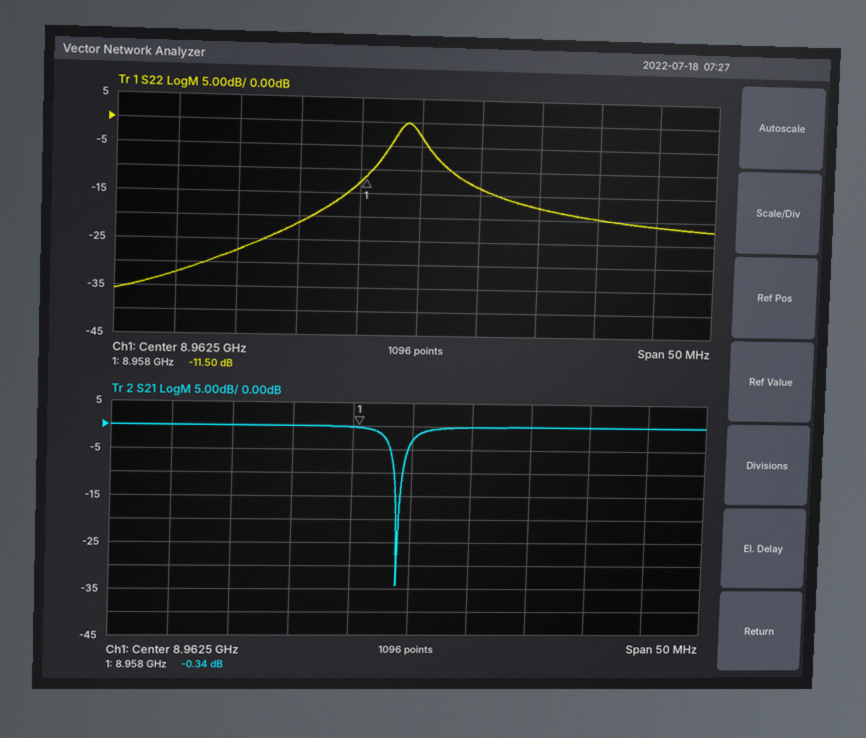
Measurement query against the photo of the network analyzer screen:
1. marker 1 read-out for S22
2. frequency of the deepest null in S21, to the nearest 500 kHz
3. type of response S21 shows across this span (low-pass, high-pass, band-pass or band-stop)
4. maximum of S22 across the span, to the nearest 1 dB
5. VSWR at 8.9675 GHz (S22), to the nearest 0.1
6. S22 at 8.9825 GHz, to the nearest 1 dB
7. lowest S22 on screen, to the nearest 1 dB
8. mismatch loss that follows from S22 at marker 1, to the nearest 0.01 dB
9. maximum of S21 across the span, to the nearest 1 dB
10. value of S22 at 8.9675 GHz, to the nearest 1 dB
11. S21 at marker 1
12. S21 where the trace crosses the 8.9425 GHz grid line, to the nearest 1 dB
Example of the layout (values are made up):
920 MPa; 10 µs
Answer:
-11.50 dB; 8.9615 GHz; band-stop; 0 dB; 1.5; -21 dB; -36 dB; 0.32 dB; 0 dB; -14 dB; -0.34 dB; 0 dB
